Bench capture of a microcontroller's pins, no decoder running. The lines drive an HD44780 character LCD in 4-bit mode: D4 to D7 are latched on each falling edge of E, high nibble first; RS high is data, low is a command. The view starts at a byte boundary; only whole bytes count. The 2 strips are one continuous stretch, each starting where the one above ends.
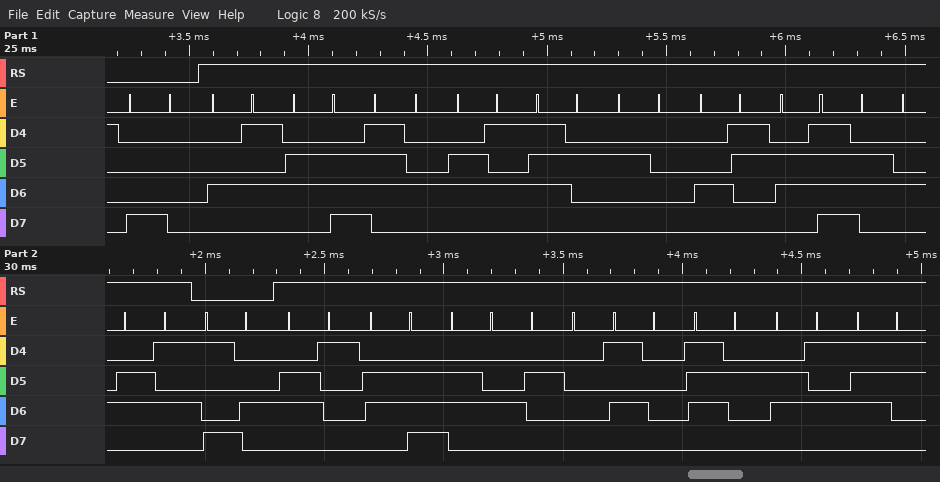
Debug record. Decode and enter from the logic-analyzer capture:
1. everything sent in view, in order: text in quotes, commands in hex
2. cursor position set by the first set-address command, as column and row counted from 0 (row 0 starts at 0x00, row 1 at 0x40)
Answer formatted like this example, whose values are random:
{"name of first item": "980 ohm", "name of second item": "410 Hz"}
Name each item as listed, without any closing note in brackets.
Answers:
{"everything sent in view, in order: text in quotes, commands in hex": "0x80 \"Enter Code\" 0x94 \"and Pres\"", "cursor position set by the first set-address command, as column and row counted from 0": "column 0, row 0"}
